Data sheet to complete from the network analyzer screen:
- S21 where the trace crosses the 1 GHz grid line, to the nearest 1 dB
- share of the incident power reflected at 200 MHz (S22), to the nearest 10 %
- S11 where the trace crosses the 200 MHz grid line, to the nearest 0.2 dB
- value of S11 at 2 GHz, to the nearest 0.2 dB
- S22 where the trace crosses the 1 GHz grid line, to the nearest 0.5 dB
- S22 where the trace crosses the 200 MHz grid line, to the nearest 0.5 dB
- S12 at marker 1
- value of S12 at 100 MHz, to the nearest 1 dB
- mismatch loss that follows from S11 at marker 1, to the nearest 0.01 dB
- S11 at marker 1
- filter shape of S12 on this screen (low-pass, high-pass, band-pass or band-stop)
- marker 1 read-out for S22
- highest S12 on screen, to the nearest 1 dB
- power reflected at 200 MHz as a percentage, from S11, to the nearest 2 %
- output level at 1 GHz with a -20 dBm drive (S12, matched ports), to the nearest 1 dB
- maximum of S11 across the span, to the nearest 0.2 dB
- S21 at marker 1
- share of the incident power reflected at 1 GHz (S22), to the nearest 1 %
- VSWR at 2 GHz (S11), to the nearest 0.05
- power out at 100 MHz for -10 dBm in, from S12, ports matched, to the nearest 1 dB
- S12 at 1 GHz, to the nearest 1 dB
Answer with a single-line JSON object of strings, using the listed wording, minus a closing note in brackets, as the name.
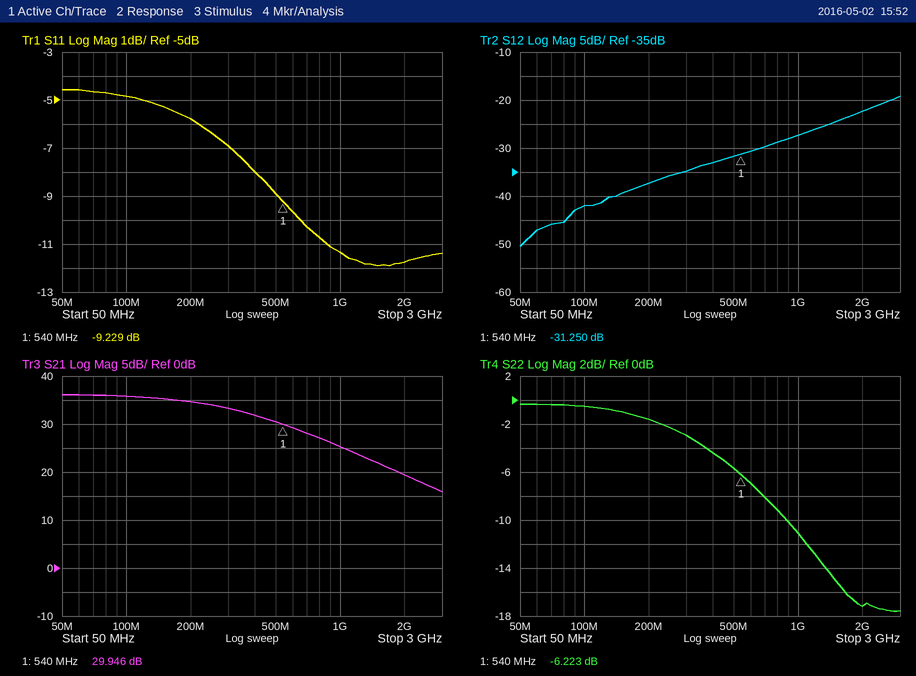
{"S21 where the trace crosses the 1 GHz grid line, to the nearest 1 dB": "25 dB", "share of the incident power reflected at 200 MHz (S22), to the nearest 10 %": "70 %", "S11 where the trace crosses the 200 MHz grid line, to the nearest 0.2 dB": "-5.8 dB", "value of S11 at 2 GHz, to the nearest 0.2 dB": "-11.8 dB", "S22 where the trace crosses the 1 GHz grid line, to the nearest 0.5 dB": "-11.0 dB", "S22 where the trace crosses the 200 MHz grid line, to the nearest 0.5 dB": "-1.5 dB", "S12 at marker 1": "-31.250 dB", "value of S12 at 100 MHz, to the nearest 1 dB": "-42 dB", "mismatch loss that follows from S11 at marker 1, to the nearest 0.01 dB": "0.55 dB", "S11 at marker 1": "-9.229 dB", "filter shape of S12 on this screen": "high-pass", "marker 1 read-out for S22": "-6.223 dB", "highest S12 on screen, to the nearest 1 dB": "-19 dB", "power reflected at 200 MHz as a percentage, from S11, to the nearest 2 %": "26 %", "output level at 1 GHz with a -20 dBm drive (S12, matched ports), to the nearest 1 dB": "-47 dBm", "maximum of S11 across the span, to the nearest 0.2 dB": "-4.6 dB", "S21 at marker 1": "29.946 dB", "share of the incident power reflected at 1 GHz (S22), to the nearest 1 %": "8 %", "VSWR at 2 GHz (S11), to the nearest 0.05": "1.70", "power out at 100 MHz for -10 dBm in, from S12, ports matched, to the nearest 1 dB": "-52 dBm", "S12 at 1 GHz, to the nearest 1 dB": "-27 dB"}
